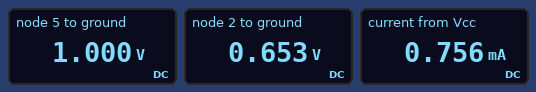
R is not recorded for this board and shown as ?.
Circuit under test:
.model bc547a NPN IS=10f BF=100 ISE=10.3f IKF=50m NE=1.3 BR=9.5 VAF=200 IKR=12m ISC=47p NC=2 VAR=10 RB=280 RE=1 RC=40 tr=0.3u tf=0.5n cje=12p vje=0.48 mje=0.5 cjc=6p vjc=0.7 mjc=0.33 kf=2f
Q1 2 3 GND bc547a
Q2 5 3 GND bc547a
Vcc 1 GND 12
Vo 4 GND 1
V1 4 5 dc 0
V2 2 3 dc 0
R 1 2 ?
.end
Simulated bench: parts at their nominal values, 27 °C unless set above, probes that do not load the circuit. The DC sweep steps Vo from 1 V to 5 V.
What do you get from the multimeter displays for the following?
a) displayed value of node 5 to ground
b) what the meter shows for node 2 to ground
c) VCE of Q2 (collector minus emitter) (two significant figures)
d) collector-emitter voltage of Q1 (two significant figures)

1.000 V
0.653 V
1.0 V
650 mV
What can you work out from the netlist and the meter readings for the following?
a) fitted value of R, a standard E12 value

15 kΩ
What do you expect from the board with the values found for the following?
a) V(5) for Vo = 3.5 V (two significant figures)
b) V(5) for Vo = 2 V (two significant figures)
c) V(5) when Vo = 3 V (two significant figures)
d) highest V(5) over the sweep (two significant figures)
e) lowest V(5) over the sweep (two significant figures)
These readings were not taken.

3.5 V
2.0 V
3.0 V
5.0 V
1.0 V
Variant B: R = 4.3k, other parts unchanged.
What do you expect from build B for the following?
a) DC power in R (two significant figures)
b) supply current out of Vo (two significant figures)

30 mW
2.6 mA
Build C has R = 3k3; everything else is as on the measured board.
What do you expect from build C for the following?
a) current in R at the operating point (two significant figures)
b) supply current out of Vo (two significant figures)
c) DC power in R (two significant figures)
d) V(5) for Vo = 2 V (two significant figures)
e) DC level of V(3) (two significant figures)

3.4 mA
3.3 mA
39 mW
2.0 V
710 mV
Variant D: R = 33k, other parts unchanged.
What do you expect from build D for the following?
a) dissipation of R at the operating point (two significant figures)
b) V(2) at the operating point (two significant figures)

3.9 mW
630 mV
